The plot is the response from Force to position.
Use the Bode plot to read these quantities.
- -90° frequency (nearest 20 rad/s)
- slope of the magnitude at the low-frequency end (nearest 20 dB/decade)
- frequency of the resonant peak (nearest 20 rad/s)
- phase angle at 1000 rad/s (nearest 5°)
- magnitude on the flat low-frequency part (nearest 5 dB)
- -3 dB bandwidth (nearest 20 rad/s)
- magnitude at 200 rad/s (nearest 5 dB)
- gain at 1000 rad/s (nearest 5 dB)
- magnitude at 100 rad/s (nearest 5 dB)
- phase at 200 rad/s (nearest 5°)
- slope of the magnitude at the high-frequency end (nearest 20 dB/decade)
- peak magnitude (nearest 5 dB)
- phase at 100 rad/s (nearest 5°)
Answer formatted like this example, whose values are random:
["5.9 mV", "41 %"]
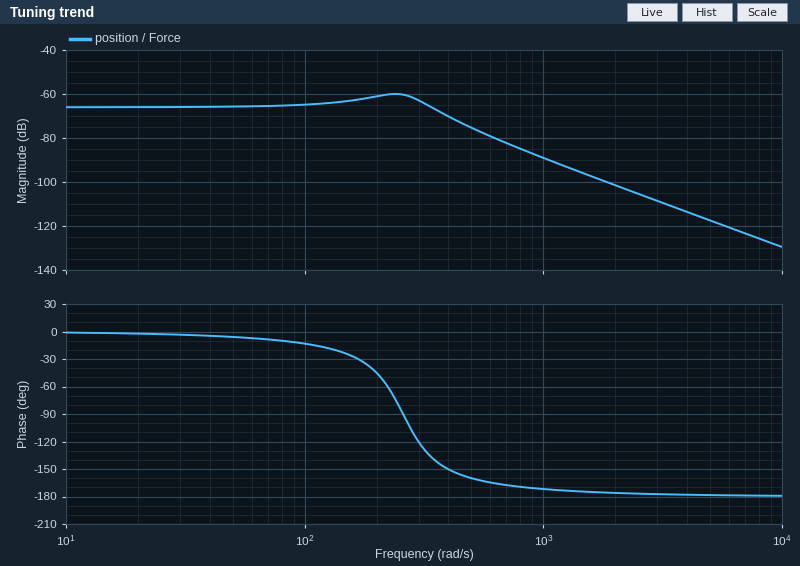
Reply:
["260 rad/s", "0 dB/decade", "240 rad/s", "-170°", "-65 dB", "380 rad/s", "-60 dB", "-90 dB", "-65 dB", "-45°", "-40 dB/decade", "-60 dB", "-15°"]
